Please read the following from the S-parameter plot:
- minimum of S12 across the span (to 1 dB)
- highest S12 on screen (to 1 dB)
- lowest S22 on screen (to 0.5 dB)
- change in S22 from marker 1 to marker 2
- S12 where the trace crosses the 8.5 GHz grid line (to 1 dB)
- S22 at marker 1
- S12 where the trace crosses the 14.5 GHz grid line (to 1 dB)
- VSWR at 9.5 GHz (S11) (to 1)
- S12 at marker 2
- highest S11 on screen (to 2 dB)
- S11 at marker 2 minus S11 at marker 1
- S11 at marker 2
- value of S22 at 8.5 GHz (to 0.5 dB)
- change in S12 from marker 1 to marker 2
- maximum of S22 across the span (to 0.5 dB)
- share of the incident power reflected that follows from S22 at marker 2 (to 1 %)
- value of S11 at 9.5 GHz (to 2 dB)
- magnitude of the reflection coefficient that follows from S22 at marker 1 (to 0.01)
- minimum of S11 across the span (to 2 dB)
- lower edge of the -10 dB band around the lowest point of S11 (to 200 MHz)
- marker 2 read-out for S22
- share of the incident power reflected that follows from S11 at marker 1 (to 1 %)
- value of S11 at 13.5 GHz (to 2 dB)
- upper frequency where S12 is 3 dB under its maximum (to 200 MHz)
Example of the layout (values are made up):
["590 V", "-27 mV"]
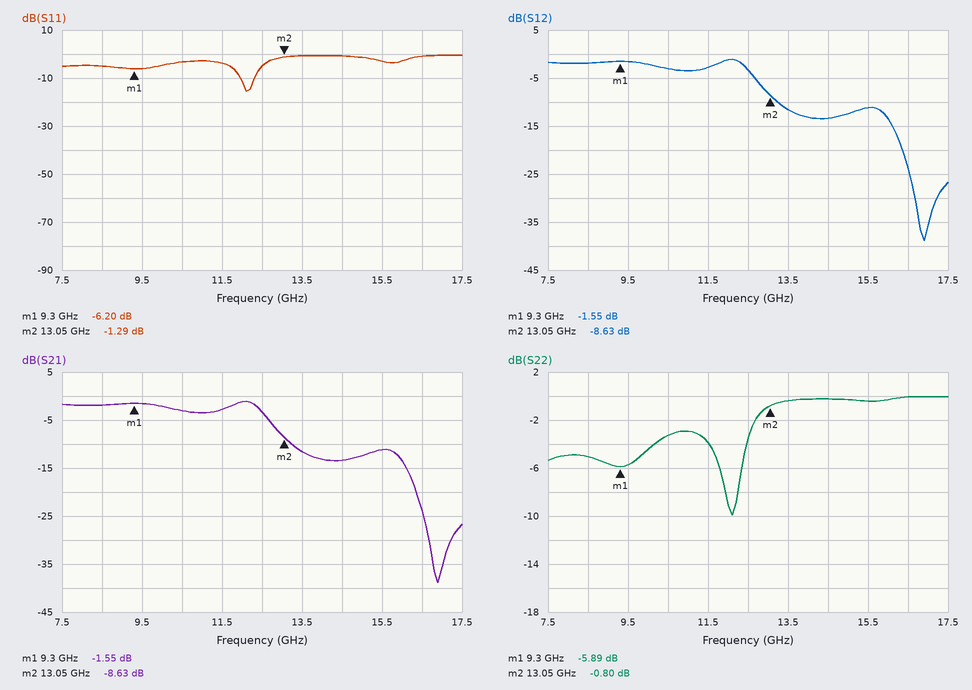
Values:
["-39 dB", "-1 dB", "-10.0 dB", "5.09 dB", "-2 dB", "-5.89 dB", "-13 dB", "3", "-8.63 dB", "0 dB", "4.91 dB", "-1.29 dB", "-5.0 dB", "-7.08 dB", "0.0 dB", "83 %", "-6 dB", "0.51", "-16 dB", "12.0 GHz", "-0.80 dB", "24 %", "0 dB", "12.6 GHz"]
